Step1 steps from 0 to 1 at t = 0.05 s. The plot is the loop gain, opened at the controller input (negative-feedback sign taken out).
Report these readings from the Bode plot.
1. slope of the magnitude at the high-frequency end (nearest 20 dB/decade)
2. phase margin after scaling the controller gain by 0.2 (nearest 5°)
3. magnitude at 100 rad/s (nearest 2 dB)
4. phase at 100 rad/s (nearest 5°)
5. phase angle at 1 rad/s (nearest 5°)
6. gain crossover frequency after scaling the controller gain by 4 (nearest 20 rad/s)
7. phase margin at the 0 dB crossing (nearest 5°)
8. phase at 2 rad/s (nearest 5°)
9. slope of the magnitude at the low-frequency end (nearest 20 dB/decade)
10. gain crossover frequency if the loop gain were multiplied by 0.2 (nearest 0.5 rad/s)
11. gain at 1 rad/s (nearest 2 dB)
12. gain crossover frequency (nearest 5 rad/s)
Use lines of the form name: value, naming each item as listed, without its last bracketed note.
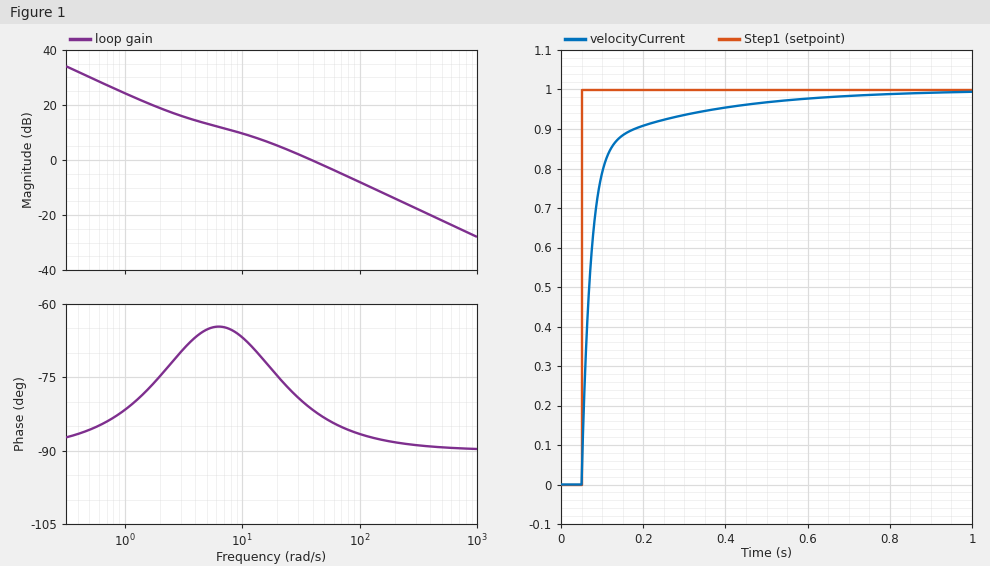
slope of the magnitude at the high-frequency end: -20 dB/decade
phase margin after scaling the controller gain by 0.2: 115°
magnitude at 100 rad/s: -8 dB
phase at 100 rad/s: -85°
phase angle at 1 rad/s: -80°
gain crossover frequency after scaling the controller gain by 4: 160 rad/s
phase margin at the 0 dB crossing: 100°
phase at 2 rad/s: -75°
slope of the magnitude at the low-frequency end: -20 dB/decade
gain crossover frequency if the loop gain were multiplied by 0.2: 4.5 rad/s
gain at 1 rad/s: 24 dB
gain crossover frequency: 40 rad/s
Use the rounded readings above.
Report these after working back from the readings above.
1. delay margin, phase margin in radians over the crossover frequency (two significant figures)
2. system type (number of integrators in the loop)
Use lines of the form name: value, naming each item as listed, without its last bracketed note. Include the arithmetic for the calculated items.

delay margin, phase margin in radians over the crossover frequency: 100 × π / 180 / 40 = 0.044 s
system type: 1
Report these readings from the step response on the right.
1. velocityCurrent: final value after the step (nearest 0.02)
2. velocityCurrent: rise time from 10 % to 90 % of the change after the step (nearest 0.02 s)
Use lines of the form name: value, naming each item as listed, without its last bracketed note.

velocityCurrent: final value after the step: 1.00
velocityCurrent: rise time from 10 % to 90 % of the change after the step: 0.12 s
